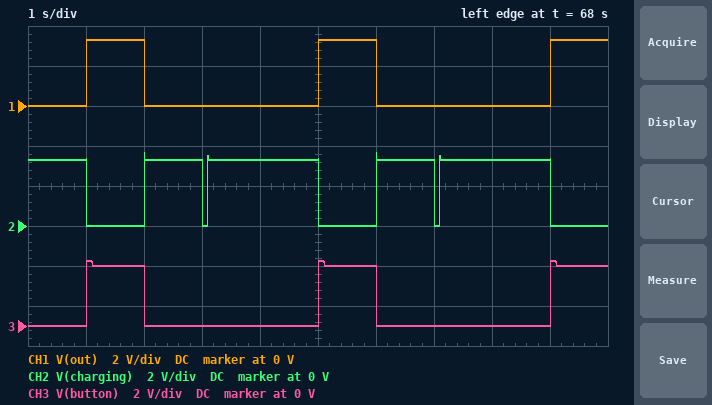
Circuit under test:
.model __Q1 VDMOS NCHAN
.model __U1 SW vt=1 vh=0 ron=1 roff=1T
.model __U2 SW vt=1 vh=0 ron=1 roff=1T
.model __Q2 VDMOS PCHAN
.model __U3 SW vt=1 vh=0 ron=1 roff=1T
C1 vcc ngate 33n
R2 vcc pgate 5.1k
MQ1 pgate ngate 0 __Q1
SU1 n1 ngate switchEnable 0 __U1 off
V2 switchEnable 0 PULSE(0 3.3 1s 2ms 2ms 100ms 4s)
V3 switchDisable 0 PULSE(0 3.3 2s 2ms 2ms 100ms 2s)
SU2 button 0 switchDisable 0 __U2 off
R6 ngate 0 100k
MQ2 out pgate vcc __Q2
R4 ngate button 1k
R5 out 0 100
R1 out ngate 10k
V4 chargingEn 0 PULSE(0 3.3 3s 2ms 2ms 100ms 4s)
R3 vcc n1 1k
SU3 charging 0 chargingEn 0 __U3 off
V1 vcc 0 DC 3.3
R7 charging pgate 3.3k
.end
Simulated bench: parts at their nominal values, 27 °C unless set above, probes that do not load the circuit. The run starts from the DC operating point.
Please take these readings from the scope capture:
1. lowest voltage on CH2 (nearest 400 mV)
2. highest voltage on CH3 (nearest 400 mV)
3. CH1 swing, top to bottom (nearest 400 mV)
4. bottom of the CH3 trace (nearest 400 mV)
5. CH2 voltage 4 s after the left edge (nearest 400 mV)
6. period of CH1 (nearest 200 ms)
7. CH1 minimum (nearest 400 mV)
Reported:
0 V
3.2 V
3.2 V
0 V
3.2 V
4.0 s
0 V
